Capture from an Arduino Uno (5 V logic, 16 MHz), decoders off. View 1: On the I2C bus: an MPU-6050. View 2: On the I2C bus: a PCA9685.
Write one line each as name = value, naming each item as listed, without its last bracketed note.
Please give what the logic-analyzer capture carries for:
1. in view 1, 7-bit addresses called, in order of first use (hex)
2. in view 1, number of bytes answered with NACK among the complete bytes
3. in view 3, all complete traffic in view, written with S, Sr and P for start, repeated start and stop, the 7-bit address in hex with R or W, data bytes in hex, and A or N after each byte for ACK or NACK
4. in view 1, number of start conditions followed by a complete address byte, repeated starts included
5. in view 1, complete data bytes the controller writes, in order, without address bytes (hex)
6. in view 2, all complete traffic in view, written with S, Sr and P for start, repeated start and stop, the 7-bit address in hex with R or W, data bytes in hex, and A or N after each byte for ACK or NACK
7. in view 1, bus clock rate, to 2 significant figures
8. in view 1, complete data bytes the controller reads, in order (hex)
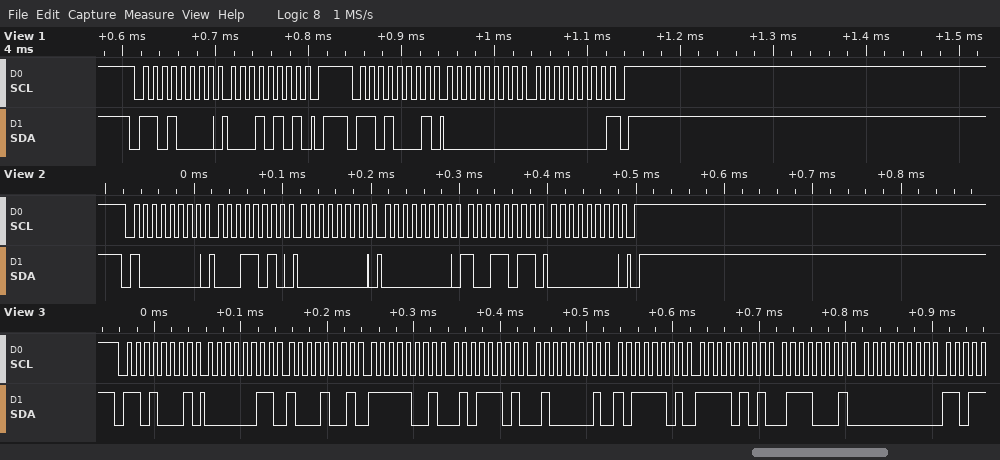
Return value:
in view 1, 7-bit addresses called, in order of first use = 0x68
in view 1, number of bytes answered with NACK among the complete bytes = 1
in view 3, all complete traffic in view, written with S, Sr and P for start, repeated start and stop, the 7-bit address in hex with R or W, data bytes in hex, and A or N after each byte for ACK or NACK = S 68R A 03 A 89 A F9 A 5D A 41 A BD A F5 A 71 A 00 A
in view 1, number of start conditions followed by a complete address byte, repeated starts included = 2
in view 1, complete data bytes the controller writes, in order, without address bytes = 15
in view 2, all complete traffic in view, written with S, Sr and P for start, repeated start and stop, the 7-bit address in hex with R or W, data bytes in hex, and A or N after each byte for ACK or NACK = S 40W A 1A A 00 A 00 A 9B A 00 A P
in view 1, bus clock rate, to 2 significant figures = 100 kHz
in view 1, complete data bytes the controller reads, in order = 00 00
